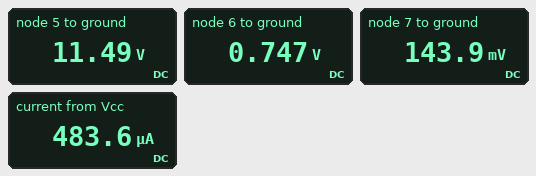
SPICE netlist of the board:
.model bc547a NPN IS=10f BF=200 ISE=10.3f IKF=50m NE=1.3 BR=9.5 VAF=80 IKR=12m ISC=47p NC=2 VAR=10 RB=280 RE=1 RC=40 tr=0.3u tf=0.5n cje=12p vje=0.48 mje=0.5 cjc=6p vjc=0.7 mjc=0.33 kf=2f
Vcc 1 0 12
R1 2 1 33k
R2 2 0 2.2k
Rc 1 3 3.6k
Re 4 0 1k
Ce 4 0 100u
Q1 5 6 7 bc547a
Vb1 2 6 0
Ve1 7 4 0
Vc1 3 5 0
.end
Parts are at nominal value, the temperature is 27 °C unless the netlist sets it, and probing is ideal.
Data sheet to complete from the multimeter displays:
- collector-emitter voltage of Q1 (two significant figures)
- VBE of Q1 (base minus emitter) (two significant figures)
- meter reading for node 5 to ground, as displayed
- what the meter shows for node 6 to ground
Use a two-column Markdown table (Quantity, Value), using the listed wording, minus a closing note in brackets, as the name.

| Quantity | Value |
|---|---|
| collector-emitter voltage of Q1 | 11 V |
| VBE of Q1 (base minus emitter) | 600 mV |
| meter reading for node 5 to ground, as displayed | 11.49 V |
| what the meter shows for node 6 to ground | 0.747 V |
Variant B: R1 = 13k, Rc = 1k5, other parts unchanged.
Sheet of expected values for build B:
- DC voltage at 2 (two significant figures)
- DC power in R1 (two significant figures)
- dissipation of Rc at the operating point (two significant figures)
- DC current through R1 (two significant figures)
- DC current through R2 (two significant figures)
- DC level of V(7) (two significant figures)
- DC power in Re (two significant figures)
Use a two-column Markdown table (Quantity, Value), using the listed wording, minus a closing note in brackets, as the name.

| Quantity | Value |
|---|---|
| DC voltage at 2 | 1.7 V |
| DC power in R1 | 8.1 mW |
| dissipation of Rc at the operating point | 1.7 mW |
| DC current through R1 | 790 µA |
| DC current through R2 | 780 µA |
| DC level of V(7) | 1.1 V |
| DC power in Re | 1.1 mW |
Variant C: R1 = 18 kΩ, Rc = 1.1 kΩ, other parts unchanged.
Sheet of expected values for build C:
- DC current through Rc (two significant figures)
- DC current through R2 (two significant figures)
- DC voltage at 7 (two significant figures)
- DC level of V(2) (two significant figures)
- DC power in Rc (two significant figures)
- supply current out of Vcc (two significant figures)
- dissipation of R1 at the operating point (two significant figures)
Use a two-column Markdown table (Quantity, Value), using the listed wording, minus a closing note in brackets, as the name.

| Quantity | Value |
|---|---|
| DC current through Rc | 650 µA |
| DC current through R2 | 590 µA |
| DC voltage at 7 | 650 mV |
| DC level of V(2) | 1.3 V |
| DC power in Rc | 460 µW |
| supply current out of Vcc | 1.2 mA |
| dissipation of R1 at the operating point | 6.4 mW |
